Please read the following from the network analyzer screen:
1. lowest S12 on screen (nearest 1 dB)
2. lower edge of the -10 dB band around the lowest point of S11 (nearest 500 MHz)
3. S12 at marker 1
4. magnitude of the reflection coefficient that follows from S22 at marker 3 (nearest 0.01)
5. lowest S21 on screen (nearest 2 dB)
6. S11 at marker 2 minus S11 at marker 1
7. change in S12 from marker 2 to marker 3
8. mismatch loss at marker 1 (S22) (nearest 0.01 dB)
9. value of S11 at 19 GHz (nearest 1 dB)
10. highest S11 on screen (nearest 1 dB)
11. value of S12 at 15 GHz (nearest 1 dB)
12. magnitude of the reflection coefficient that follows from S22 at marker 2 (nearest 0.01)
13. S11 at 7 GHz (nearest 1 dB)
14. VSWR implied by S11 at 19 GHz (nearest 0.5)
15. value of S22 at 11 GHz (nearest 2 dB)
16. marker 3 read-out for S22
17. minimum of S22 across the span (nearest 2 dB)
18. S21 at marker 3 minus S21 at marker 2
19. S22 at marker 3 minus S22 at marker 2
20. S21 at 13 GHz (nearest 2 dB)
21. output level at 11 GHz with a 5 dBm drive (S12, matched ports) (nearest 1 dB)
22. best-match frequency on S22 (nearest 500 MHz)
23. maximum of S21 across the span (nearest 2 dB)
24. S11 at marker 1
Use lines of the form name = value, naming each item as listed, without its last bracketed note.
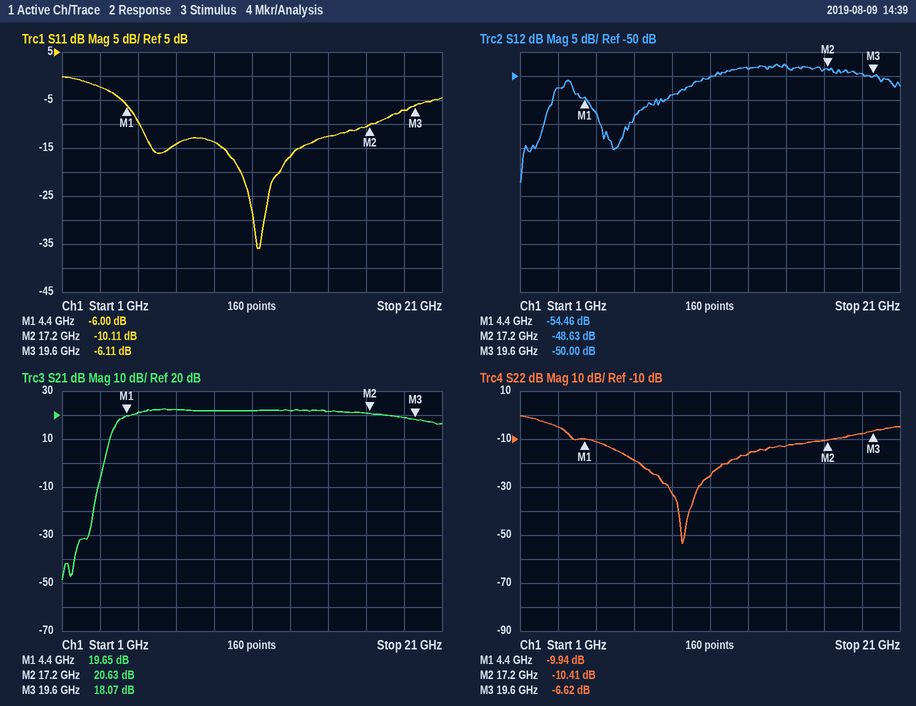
lowest S12 on screen = -72 dB
lower edge of the -10 dB band around the lowest point of S11 = 5.0 GHz
S12 at marker 1 = -54.46 dB
magnitude of the reflection coefficient that follows from S22 at marker 3 = 0.47
lowest S21 on screen = -48 dB
S11 at marker 2 minus S11 at marker 1 = -4.11 dB
change in S12 from marker 2 to marker 3 = -1.37 dB
mismatch loss at marker 1 (S22) = 0.46 dB
value of S11 at 19 GHz = -7 dB
highest S11 on screen = 0 dB
value of S12 at 15 GHz = -48 dB
magnitude of the reflection coefficient that follows from S22 at marker 2 = 0.30
S11 at 7 GHz = -14 dB
VSWR implied by S11 at 19 GHz = 2.5
value of S22 at 11 GHz = -26 dB
marker 3 read-out for S22 = -6.62 dB
minimum of S22 across the span = -54 dB
S21 at marker 3 minus S21 at marker 2 = -2.56 dB
S22 at marker 3 minus S22 at marker 2 = 3.79 dB
S21 at 13 GHz = 22 dB
output level at 11 GHz with a 5 dBm drive (S12, matched ports) = -45 dBm
best-match frequency on S22 = 9.5 GHz
maximum of S21 across the span = 22 dB
S11 at marker 1 = -6.00 dB
